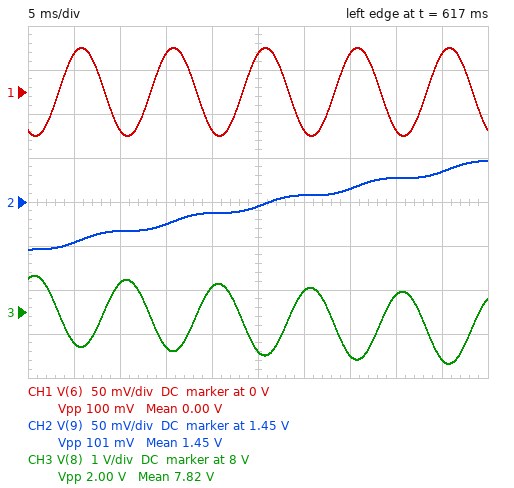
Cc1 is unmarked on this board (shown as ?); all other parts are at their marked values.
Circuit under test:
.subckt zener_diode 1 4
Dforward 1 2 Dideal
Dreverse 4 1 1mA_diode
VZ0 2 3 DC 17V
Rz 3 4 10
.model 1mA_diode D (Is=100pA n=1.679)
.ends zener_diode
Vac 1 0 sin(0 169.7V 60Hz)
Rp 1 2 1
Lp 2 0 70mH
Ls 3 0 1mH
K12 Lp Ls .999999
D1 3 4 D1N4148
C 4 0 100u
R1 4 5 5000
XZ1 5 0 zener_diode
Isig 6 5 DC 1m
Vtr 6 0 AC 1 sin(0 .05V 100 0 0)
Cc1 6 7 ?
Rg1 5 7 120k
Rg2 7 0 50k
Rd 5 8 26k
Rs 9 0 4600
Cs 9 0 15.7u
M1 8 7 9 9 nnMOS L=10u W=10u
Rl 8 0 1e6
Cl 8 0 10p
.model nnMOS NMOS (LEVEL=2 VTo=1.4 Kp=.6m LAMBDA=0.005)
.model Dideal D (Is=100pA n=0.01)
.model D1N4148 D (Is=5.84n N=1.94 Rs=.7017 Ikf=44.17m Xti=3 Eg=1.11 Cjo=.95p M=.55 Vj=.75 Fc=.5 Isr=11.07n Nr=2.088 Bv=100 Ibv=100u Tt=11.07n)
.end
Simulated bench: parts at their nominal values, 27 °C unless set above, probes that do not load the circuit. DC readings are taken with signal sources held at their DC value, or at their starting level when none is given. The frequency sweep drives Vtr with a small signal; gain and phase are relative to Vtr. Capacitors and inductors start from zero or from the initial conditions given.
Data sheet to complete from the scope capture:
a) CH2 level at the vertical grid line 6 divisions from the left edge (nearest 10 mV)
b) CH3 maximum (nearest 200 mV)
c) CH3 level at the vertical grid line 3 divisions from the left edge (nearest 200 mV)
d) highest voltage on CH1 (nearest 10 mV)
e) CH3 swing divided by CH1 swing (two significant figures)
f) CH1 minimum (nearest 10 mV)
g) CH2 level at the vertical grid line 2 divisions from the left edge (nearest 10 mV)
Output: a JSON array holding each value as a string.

["1.46 V", "8.8 V", "7.2 V", "50 mV", "20", "-50 mV", "1.42 V"]
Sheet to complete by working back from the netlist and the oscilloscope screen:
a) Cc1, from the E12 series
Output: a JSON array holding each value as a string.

["12 µF"]
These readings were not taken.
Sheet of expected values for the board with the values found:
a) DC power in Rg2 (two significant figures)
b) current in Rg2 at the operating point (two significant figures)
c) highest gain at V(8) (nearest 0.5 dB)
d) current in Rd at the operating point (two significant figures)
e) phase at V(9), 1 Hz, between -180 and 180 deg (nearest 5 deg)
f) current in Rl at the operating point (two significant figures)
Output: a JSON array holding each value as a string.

["500 µW", "100 µA", "25.5 dB", "510 µA", "15 deg", "3.8 µA"]
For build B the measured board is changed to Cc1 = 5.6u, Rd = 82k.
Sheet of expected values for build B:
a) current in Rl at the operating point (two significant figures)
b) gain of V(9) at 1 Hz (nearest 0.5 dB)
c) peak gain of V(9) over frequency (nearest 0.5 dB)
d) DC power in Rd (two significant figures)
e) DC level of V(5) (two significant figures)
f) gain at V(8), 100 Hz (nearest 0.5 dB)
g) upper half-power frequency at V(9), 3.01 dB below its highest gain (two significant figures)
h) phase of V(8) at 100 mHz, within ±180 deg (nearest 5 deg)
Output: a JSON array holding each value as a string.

["1.0 µA", "-54.5 dB", "-54.0 dB", "3.1 mW", "17 V", "-26.5 dB", "3.7 Hz", "-95 deg"]
